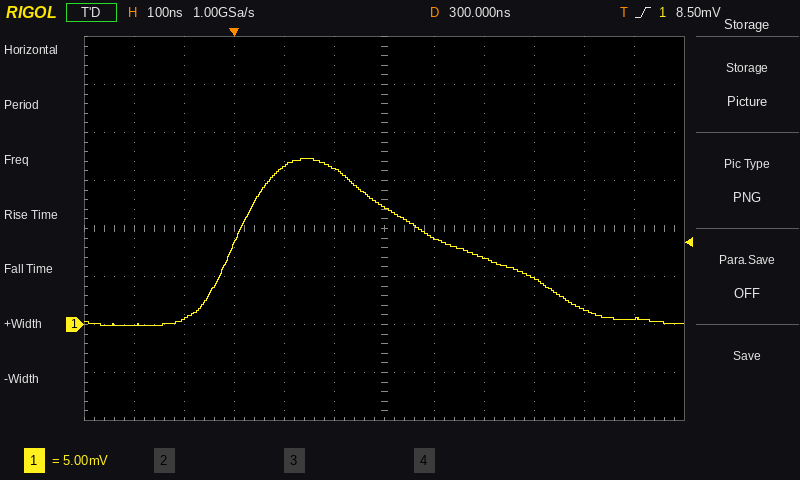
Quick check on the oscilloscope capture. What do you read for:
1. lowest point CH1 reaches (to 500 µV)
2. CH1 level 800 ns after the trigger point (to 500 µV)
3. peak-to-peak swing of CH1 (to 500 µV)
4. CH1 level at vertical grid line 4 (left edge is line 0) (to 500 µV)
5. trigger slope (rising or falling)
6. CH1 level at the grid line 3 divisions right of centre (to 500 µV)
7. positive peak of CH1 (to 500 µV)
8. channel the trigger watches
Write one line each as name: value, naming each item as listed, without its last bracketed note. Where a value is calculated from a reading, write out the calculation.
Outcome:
lowest point CH1 reaches: 0.0 mV
CH1 level 800 ns after the trigger point: 500 µV
peak-to-peak swing of CH1: 17.5 mV − (0.0 mV) = 17.5 mV
CH1 level at vertical grid line 4 (left edge is line 0): 16.5 mV
trigger slope: rising
CH1 level at the grid line 3 divisions right of centre: 5.0 mV
positive peak of CH1: 17.5 mV
channel the trigger watches: CH1
